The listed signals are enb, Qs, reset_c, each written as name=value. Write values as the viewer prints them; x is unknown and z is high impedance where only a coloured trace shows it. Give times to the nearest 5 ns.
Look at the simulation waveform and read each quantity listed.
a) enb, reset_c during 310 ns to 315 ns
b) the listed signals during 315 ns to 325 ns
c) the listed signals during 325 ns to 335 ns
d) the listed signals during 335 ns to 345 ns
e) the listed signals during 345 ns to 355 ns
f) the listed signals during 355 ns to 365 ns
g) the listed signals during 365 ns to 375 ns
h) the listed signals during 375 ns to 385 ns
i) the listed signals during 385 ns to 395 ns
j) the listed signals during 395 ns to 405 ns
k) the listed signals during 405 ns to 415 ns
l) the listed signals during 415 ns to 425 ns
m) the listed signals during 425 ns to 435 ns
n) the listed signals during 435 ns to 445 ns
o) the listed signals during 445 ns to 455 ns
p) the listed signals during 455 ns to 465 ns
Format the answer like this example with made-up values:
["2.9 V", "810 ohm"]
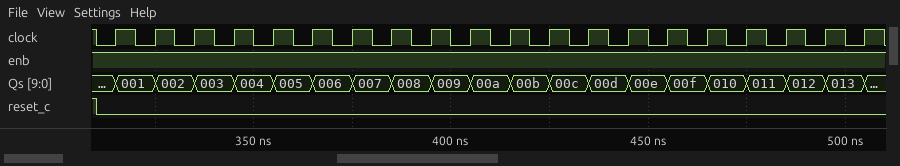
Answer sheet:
["enb=1, reset_c=0", "enb=1, Qs=001, reset_c=0", "enb=1, Qs=002, reset_c=0", "enb=1, Qs=003, reset_c=0", "enb=1, Qs=004, reset_c=0", "enb=1, Qs=005, reset_c=0", "enb=1, Qs=006, reset_c=0", "enb=1, Qs=007, reset_c=0", "enb=1, Qs=008, reset_c=0", "enb=1, Qs=009, reset_c=0", "enb=1, Qs=00a, reset_c=0", "enb=1, Qs=00b, reset_c=0", "enb=1, Qs=00c, reset_c=0", "enb=1, Qs=00d, reset_c=0", "enb=1, Qs=00e, reset_c=0", "enb=1, Qs=00f, reset_c=0"]
